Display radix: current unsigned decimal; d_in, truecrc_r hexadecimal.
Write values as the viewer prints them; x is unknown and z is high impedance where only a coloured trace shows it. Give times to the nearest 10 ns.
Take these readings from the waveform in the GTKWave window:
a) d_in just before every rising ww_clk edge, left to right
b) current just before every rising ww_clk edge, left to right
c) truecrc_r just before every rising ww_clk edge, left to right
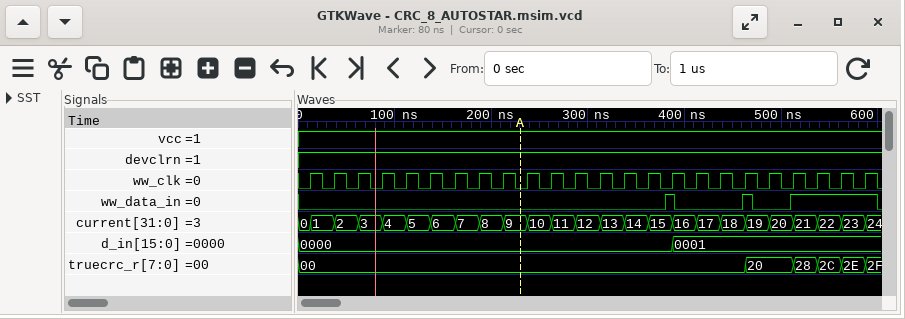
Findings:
0000, 0000, 0000, 0000, 0000, 0000, 0000, 0000, 0000, 0000, 0000, 0000, 0000, 0000, 0000, 0000, 0001, 0001, 0001, 0001, 0001, 0001, 0001, 0001
0, 1, 2, 3, 4, 5, 6, 7, 8, 9, 10, 11, 12, 13, 14, 15, 16, 17, 18, 19, 20, 21, 22, 23
00, 00, 00, 00, 00, 00, 00, 00, 00, 00, 00, 00, 00, 00, 00, 00, 00, 00, 00, 20, 20, 28, 2C, 2E
